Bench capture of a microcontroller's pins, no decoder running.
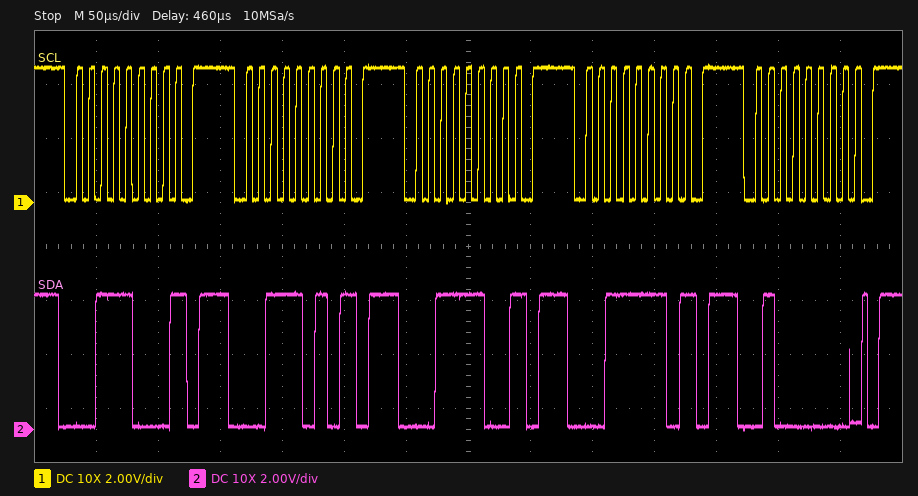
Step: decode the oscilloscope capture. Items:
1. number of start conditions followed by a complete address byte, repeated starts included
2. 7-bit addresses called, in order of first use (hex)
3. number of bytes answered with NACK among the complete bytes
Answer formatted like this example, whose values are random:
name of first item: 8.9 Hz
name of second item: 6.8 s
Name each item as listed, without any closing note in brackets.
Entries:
number of start conditions followed by a complete address byte, repeated starts included: 5
7-bit addresses called, in order of first use: 0x1C 0x1D 0x1E 0x1F 0x20
number of bytes answered with NACK among the complete bytes: 4
